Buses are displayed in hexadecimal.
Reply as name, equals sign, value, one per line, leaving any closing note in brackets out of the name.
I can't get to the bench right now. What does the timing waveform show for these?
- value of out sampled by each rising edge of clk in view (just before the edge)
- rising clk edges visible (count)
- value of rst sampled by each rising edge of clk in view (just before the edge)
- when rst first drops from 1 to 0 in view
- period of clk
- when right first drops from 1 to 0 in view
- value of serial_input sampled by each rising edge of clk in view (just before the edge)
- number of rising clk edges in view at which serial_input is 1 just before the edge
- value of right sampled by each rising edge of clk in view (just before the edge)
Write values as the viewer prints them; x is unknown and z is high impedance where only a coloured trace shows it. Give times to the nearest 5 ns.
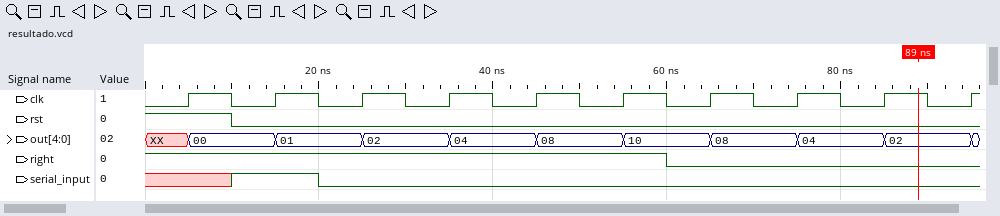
value of out sampled by each rising edge of clk in view = XX, 00, 01, 02, 04, 08, 10, 08, 04, 02
rising clk edges visible = 10
value of rst sampled by each rising edge of clk in view = 1 0 0 0 0 0 0 0 0 0
when rst first drops from 1 to 0 in view = 10 ns
period of clk = 10 ns
when right first drops from 1 to 0 in view = 60 ns
value of serial_input sampled by each rising edge of clk in view = x 1 0 0 0 0 0 0 0 0
number of rising clk edges in view at which serial_input is 1 just before the edge = 1
value of right sampled by each rising edge of clk in view = 1 1 1 1 1 1 0 0 0 0
